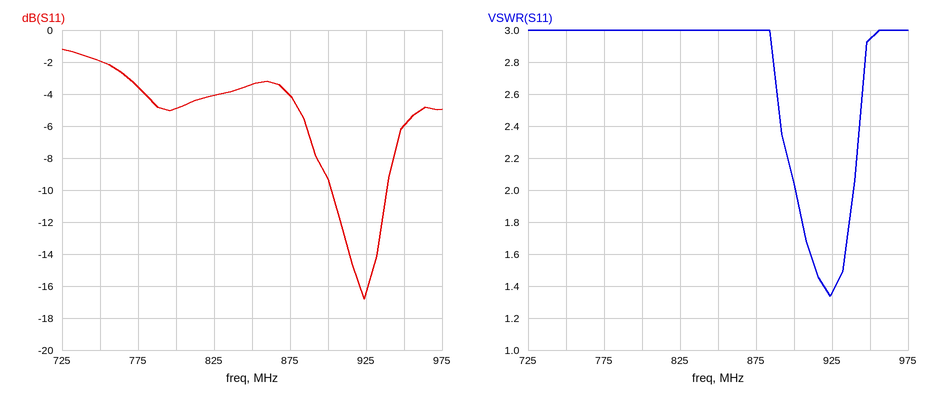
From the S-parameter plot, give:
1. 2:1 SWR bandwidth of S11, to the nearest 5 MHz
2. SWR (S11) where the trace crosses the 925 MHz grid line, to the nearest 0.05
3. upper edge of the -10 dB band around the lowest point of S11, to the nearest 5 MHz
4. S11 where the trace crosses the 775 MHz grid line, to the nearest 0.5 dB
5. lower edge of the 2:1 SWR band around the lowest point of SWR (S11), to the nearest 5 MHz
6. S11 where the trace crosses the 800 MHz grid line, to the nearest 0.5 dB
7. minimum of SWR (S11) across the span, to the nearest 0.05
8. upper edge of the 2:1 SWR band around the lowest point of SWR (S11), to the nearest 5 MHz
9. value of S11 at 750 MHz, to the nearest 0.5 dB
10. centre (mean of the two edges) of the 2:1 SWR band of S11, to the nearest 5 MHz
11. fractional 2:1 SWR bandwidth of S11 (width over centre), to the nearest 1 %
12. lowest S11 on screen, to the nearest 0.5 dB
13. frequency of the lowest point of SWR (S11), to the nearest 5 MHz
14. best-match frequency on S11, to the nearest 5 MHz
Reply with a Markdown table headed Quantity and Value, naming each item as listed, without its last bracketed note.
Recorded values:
| Quantity | Value |
|---|---|
| 2:1 SWR bandwidth of S11, to the nearest 5 MHz | 40 MHz |
| SWR (S11) where the trace crosses the 925 MHz grid line, to the nearest 0.05 | 1.35 |
| upper edge of the -10 dB band around the lowest point of S11, to the nearest 5 MHz | 940 MHz |
| S11 where the trace crosses the 775 MHz grid line, to the nearest 0.5 dB | -3.5 dB |
| lower edge of the 2:1 SWR band around the lowest point of SWR (S11), to the nearest 5 MHz | 900 MHz |
| S11 where the trace crosses the 800 MHz grid line, to the nearest 0.5 dB | -5.0 dB |
| minimum of SWR (S11) across the span, to the nearest 0.05 | 1.35 |
| upper edge of the 2:1 SWR band around the lowest point of SWR (S11), to the nearest 5 MHz | 940 MHz |
| value of S11 at 750 MHz, to the nearest 0.5 dB | -2.0 dB |
| centre (mean of the two edges) of the 2:1 SWR band of S11, to the nearest 5 MHz | 920 MHz |
| fractional 2:1 SWR bandwidth of S11 (width over centre), to the nearest 1 % | 4 % |
| lowest S11 on screen, to the nearest 0.5 dB | -17.0 dB |
| frequency of the lowest point of SWR (S11), to the nearest 5 MHz | 925 MHz |
| best-match frequency on S11, to the nearest 5 MHz | 925 MHz |
